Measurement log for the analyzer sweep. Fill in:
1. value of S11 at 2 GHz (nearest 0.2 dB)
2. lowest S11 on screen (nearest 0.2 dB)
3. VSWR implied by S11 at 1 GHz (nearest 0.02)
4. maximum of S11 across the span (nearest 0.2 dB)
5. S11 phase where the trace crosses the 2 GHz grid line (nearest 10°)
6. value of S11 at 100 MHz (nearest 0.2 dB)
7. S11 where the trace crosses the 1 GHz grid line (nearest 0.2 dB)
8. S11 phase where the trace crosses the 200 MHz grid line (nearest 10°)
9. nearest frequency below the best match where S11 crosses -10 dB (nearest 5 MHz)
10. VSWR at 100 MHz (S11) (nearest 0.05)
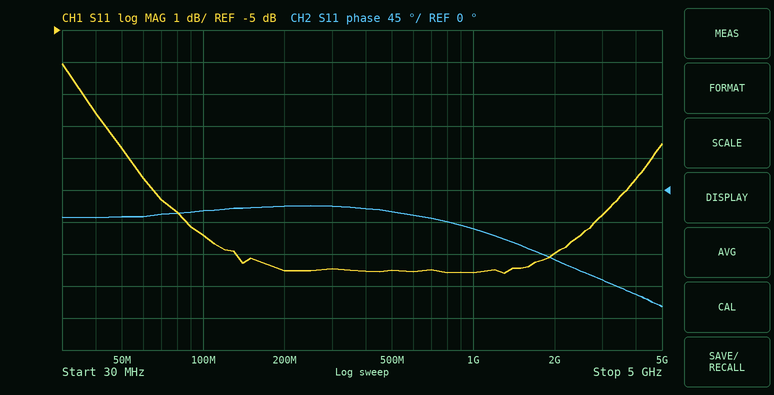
-12.0 dB
-12.6 dB
1.62
-6.0 dB
-100°
-11.4 dB
-12.6 dB
-20°
65 MHz
1.75
